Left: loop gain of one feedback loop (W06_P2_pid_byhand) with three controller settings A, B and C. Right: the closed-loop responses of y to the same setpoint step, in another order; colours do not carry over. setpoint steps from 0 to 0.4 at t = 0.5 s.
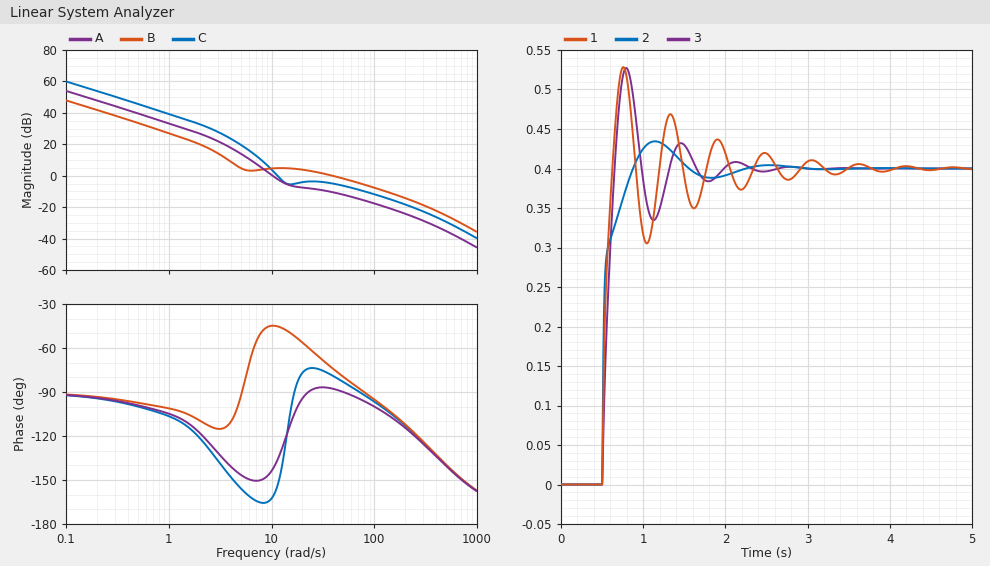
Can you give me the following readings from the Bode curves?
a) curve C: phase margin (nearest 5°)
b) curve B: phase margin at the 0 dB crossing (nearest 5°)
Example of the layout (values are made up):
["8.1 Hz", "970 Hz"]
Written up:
["25°", "105°"]
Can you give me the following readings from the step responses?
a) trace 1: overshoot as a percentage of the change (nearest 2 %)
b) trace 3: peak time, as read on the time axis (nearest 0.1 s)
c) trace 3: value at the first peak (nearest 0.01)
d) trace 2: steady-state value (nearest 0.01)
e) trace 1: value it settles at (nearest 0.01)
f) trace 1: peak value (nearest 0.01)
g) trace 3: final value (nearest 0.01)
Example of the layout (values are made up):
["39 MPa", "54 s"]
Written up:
["32 %", "0.8 s", "0.53", "0.40", "0.40", "0.53", "0.40"]
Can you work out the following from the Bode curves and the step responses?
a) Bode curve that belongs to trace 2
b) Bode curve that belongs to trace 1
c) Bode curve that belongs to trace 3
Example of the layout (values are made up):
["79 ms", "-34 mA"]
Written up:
["B", "C", "A"]
